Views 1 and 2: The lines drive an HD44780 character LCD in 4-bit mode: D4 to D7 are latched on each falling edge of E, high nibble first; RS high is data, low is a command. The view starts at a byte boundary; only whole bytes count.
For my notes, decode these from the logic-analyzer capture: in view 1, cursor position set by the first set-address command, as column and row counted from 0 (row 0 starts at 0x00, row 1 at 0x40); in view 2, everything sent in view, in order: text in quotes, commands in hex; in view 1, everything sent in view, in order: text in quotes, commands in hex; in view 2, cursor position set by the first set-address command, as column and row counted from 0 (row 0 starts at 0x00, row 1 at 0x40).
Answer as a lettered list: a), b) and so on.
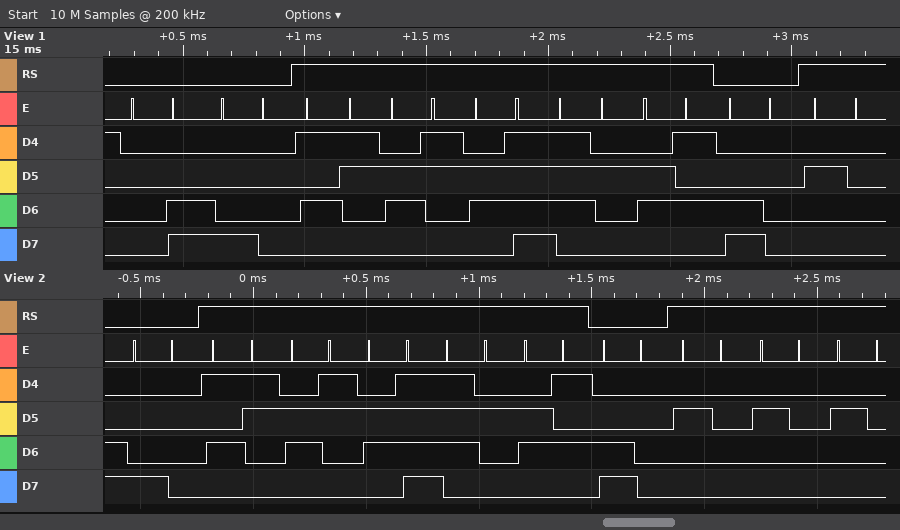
a) column 0, row 0
b) 0x80 "Score" 0xC0 "   "
c) 0x0C 0x80 "Score" 0xC0 " "
d) column 0, row 0
